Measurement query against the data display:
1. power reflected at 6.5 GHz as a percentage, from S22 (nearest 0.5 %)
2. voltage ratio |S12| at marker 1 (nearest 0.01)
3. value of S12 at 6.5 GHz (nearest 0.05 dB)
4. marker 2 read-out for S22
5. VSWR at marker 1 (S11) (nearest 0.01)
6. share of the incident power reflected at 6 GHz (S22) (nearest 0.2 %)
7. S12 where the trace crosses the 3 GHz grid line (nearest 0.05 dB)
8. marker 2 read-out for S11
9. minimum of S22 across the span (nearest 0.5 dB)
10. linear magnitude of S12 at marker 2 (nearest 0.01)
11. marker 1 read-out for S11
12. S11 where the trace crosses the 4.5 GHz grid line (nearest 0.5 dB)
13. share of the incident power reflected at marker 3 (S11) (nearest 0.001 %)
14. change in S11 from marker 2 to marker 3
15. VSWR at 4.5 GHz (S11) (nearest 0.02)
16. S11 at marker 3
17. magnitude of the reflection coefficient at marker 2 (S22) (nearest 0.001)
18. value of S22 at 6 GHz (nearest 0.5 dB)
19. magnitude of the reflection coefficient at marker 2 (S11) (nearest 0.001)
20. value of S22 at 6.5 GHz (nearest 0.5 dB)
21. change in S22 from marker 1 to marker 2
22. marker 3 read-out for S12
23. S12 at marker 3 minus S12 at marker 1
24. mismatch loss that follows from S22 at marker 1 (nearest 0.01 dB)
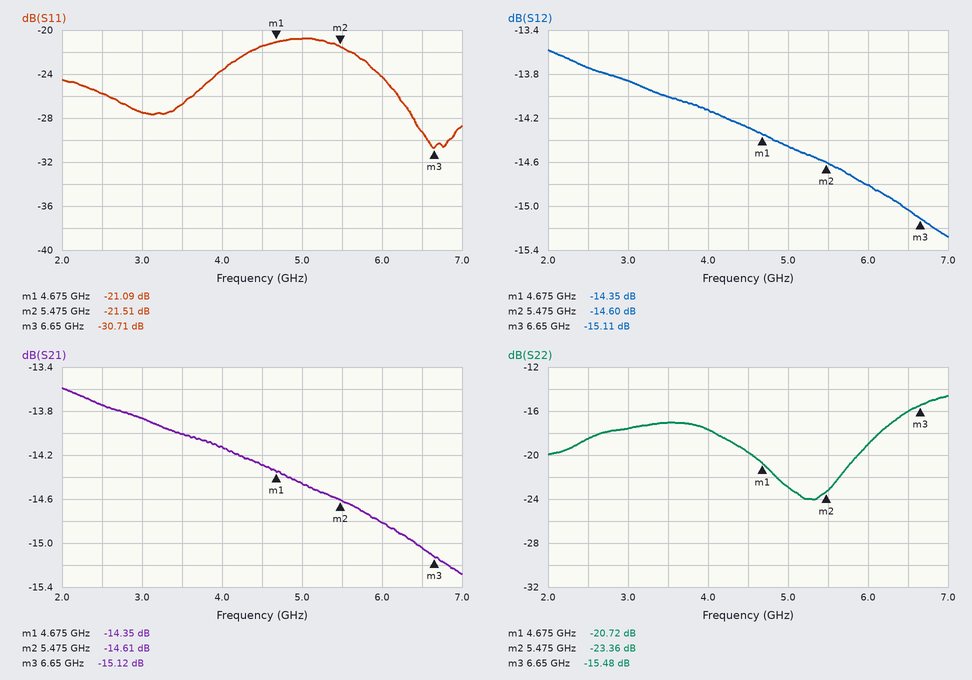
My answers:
2.5 %
0.19
-15.05 dB
-23.36 dB
1.19
1.2 %
-13.85 dB
-21.51 dB
-24.0 dB
0.19
-21.09 dB
-21.5 dB
0.085 %
-9.20 dB
1.18
-30.71 dB
0.068
-19.0 dB
0.084
-16.0 dB
-2.64 dB
-15.11 dB
-0.76 dB
0.04 dB
